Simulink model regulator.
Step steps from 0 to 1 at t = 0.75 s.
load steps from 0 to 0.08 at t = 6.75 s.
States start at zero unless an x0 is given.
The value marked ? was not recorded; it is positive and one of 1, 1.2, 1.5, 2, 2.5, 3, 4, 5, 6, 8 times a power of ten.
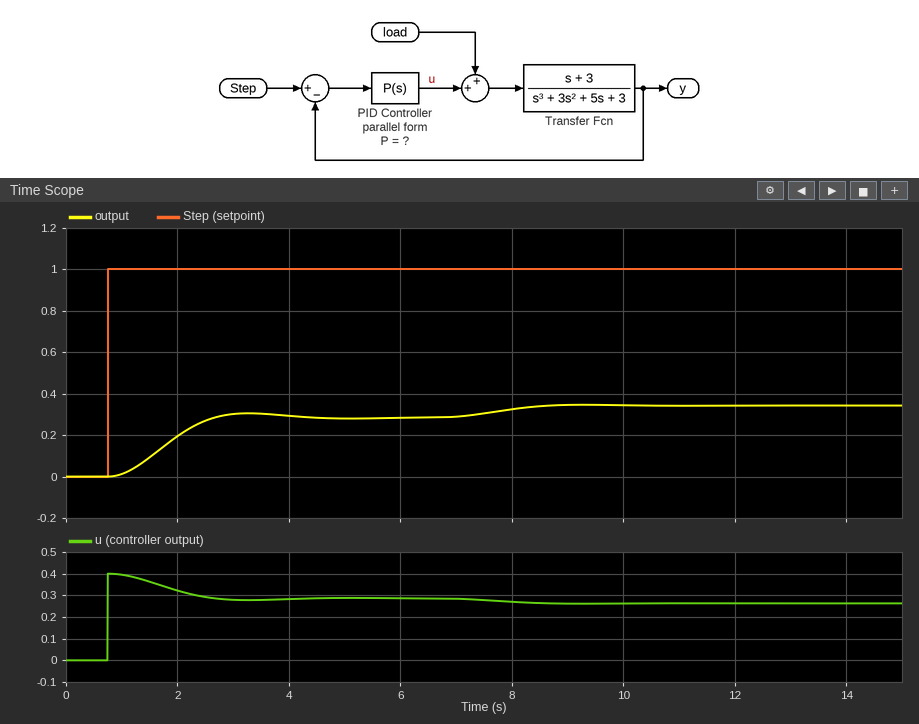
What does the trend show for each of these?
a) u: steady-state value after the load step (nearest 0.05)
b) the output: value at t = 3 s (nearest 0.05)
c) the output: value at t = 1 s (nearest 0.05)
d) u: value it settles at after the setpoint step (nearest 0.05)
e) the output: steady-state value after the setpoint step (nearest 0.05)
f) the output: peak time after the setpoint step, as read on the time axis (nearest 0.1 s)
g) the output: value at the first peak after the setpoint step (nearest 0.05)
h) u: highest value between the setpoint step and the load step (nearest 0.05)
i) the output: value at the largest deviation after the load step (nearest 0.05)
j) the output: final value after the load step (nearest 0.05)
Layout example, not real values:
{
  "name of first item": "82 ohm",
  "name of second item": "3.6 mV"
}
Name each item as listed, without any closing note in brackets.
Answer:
{
  "u: steady-state value after the load step": "0.25",
  "the output: value at t = 3 s": "0.30",
  "the output: value at t = 1 s": "0.00",
  "u: value it settles at after the setpoint step": "0.30",
  "the output: steady-state value after the setpoint step": "0.30",
  "the output: peak time after the setpoint step, as read on the time axis": "3.3 s",
  "the output: value at the first peak after the setpoint step": "0.30",
  "u: highest value between the setpoint step and the load step": "0.40",
  "the output: value at the largest deviation after the load step": "0.35",
  "the output: final value after the load step": "0.35"
}
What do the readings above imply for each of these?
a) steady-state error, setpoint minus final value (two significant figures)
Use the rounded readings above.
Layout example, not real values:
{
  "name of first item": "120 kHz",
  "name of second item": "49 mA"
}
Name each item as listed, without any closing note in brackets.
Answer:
{
  "steady-state error, setpoint minus final value": "0.70"
}
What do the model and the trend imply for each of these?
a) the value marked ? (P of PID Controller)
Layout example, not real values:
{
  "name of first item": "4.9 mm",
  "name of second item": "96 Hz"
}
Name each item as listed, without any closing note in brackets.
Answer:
{
  "the value marked ?": "0.4"
}
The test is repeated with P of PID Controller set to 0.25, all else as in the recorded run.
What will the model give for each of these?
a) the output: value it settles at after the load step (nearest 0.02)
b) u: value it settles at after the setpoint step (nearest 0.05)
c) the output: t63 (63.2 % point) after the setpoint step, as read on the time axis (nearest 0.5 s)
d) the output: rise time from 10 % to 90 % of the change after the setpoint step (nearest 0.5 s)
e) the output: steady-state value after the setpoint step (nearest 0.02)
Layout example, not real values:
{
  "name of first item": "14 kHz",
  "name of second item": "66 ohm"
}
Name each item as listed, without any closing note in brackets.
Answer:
{
  "the output: value it settles at after the load step": "0.26",
  "u: value it settles at after the setpoint step": "0.20",
  "the output: t63 (63.2 % point) after the setpoint step, as read on the time axis": "2.0 s",
  "the output: rise time from 10 % to 90 % of the change after the setpoint step": "1.5 s",
  "the output: steady-state value after the setpoint step": "0.20"
}
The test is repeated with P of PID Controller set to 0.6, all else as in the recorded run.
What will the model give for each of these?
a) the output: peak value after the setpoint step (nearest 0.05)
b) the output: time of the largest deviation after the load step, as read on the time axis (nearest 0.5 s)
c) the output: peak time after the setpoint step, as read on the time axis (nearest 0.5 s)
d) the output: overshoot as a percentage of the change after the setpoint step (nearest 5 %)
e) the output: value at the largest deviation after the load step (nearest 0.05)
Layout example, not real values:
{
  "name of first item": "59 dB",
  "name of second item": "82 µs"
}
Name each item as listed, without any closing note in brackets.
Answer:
{
  "the output: peak value after the setpoint step": "0.40",
  "the output: time of the largest deviation after the load step, as read on the time axis": "9.0 s",
  "the output: peak time after the setpoint step, as read on the time axis": "3.0 s",
  "the output: overshoot as a percentage of the change after the setpoint step": "10 %",
  "the output: value at the largest deviation after the load step": "0.45"
}
